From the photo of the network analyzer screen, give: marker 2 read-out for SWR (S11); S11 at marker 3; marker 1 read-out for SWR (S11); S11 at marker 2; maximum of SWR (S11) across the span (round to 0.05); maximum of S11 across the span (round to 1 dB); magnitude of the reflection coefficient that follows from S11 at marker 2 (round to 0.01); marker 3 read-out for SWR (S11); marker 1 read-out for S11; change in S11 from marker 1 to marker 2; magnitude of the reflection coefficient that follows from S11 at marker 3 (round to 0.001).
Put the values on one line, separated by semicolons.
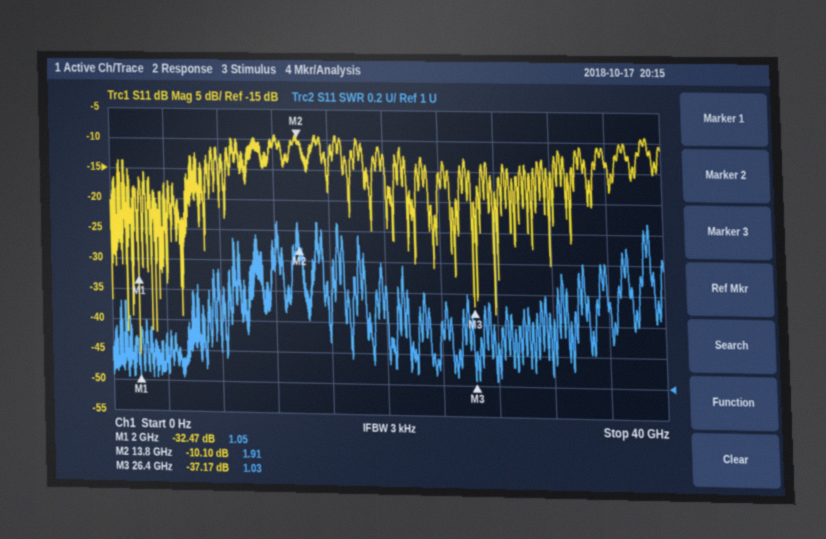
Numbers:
1.91; -37.17 dB; 1.05; -10.10 dB; 2.05; -9 dB; 0.31; 1.03; -32.47 dB; 22.37 dB; 0.014
